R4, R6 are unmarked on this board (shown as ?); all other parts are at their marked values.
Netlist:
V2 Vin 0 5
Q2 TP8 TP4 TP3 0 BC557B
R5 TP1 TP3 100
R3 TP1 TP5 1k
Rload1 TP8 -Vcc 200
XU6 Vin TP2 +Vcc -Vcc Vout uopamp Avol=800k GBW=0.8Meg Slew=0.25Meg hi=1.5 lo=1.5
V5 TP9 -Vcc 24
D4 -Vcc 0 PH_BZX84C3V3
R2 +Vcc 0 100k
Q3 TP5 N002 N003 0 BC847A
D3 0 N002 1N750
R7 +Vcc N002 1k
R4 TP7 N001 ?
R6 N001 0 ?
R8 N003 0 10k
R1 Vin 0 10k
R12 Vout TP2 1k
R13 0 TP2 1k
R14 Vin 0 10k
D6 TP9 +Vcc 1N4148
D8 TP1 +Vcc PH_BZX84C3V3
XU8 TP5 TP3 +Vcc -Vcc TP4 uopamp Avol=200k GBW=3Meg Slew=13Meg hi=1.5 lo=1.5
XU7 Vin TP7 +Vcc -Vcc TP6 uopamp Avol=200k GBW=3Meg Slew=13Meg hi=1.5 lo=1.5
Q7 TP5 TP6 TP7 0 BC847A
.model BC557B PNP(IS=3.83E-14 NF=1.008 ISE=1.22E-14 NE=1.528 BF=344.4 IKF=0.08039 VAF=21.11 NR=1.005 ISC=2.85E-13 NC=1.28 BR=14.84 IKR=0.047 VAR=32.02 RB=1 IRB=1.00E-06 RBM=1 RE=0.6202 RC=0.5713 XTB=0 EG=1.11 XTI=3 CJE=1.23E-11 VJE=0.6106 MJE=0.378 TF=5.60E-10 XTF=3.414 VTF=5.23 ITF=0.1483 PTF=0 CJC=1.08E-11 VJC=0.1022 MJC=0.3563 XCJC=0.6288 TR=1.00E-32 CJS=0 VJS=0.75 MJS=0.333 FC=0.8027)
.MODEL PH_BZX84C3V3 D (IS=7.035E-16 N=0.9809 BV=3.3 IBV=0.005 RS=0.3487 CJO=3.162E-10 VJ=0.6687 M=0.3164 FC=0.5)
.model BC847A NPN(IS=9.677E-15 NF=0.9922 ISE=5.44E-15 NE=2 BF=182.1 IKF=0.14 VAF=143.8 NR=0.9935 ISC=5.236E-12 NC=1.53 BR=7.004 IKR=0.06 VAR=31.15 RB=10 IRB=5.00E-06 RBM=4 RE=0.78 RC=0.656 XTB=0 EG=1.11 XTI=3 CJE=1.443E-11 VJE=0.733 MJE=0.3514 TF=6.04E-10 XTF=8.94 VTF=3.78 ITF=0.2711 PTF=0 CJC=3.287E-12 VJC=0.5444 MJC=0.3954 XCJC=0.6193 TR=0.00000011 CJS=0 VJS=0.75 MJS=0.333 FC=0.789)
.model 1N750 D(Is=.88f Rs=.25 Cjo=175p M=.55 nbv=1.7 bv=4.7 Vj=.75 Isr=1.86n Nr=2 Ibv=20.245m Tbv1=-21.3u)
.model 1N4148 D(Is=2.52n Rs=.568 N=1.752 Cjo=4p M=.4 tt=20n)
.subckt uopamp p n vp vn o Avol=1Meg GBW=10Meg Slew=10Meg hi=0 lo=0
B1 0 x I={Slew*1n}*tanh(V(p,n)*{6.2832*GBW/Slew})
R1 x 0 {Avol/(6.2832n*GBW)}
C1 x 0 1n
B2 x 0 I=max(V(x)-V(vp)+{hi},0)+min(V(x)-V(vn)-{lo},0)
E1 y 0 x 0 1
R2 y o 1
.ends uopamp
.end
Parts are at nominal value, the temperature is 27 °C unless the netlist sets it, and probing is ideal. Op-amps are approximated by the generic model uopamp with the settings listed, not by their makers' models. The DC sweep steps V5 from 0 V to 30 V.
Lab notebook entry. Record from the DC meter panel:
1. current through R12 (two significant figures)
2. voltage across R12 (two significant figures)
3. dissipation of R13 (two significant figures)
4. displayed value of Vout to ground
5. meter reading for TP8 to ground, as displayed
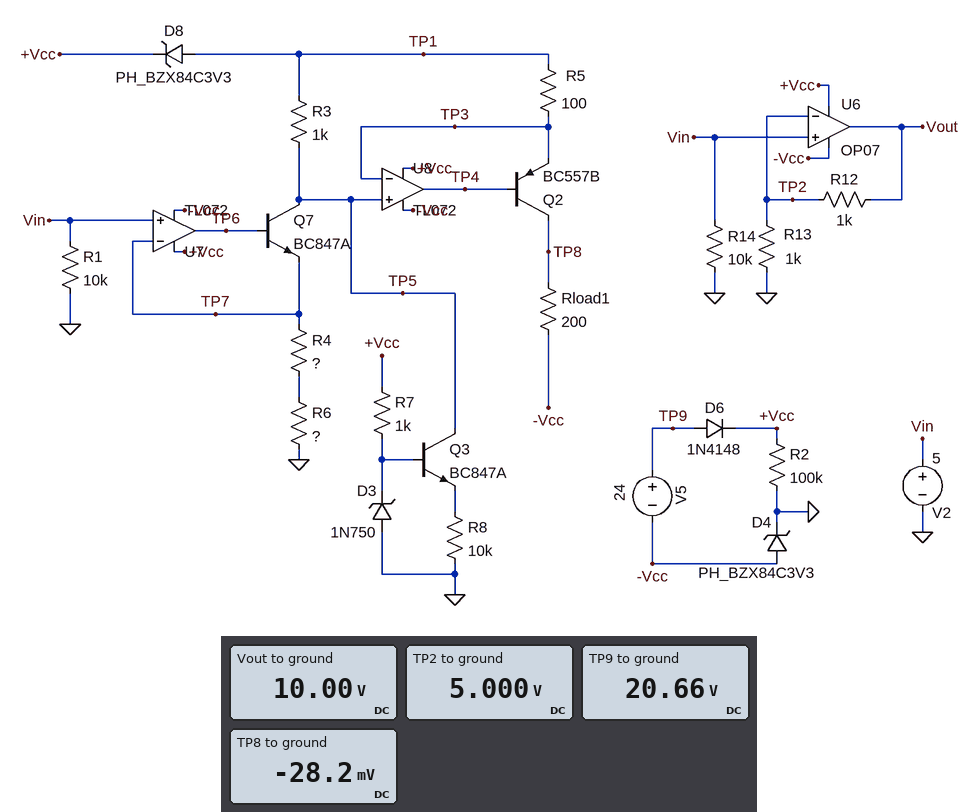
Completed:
5.0 mA
5.0 V
25 mW
10.00 V
-28.2 mV
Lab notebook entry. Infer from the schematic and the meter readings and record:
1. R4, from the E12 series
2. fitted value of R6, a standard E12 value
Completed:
3.9 kΩ
68 Ω
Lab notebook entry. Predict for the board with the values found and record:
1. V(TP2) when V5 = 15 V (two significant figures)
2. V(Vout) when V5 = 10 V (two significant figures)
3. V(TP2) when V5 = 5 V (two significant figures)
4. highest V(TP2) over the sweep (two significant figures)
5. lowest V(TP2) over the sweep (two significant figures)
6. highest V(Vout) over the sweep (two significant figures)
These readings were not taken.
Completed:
4.7 V
4.6 V
-97 mV
5.0 V
-430 mV
10 V
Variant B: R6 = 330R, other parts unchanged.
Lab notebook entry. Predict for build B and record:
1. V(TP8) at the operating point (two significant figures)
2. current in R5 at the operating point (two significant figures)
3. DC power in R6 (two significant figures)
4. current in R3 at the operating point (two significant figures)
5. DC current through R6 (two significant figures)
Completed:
-180 mV
16 mA
460 µW
1.6 mA
1.2 mA
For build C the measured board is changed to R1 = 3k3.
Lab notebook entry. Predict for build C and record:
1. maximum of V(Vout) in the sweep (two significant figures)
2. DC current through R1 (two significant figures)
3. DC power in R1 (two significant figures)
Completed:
10 V
1.5 mA
7.6 mW
